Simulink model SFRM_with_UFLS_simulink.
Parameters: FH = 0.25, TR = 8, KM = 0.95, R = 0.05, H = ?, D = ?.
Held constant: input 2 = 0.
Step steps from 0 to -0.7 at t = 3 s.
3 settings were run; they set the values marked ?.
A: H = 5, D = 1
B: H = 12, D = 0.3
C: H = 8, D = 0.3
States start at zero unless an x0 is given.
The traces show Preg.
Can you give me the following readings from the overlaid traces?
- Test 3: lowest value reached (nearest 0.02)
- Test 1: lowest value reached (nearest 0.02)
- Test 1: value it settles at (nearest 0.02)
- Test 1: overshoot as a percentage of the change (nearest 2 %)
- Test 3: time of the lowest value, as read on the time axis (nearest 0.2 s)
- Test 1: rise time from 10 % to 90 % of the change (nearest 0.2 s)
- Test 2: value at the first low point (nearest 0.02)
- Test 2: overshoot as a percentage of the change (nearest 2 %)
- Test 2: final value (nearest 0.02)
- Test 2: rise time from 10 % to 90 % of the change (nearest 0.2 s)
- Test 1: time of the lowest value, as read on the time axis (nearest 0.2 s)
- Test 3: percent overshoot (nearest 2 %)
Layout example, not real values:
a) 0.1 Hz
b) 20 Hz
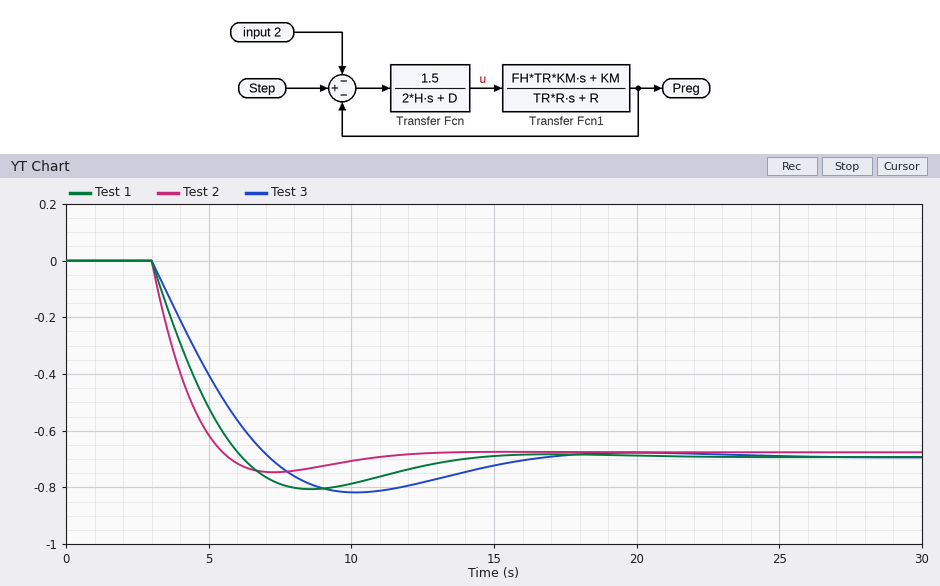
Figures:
a) -0.82
b) -0.80
c) -0.70
d) 16 %
e) 10.2 s
f) 2.4 s
g) -0.74
h) 10 %
i) -0.68
j) 1.8 s
k) 8.6 s
l) 18 %
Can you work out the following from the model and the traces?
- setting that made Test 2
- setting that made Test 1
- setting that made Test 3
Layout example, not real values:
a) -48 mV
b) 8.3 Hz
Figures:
a) A
b) C
c) B
